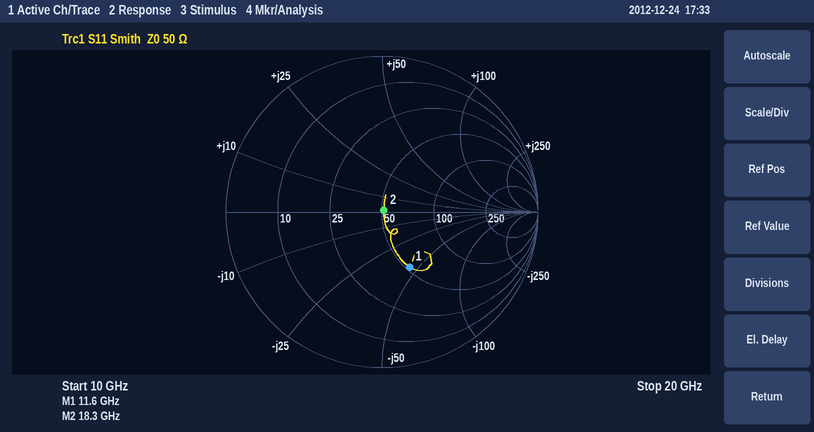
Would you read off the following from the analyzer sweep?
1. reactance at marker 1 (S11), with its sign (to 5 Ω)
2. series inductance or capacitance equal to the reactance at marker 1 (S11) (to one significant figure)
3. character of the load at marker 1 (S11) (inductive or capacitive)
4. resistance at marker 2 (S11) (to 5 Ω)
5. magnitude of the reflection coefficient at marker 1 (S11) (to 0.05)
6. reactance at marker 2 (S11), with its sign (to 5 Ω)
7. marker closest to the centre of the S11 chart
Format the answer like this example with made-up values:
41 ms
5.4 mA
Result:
-45 Ω
300 fF
capacitive
50 Ω
0.40
0 Ω
marker 2
